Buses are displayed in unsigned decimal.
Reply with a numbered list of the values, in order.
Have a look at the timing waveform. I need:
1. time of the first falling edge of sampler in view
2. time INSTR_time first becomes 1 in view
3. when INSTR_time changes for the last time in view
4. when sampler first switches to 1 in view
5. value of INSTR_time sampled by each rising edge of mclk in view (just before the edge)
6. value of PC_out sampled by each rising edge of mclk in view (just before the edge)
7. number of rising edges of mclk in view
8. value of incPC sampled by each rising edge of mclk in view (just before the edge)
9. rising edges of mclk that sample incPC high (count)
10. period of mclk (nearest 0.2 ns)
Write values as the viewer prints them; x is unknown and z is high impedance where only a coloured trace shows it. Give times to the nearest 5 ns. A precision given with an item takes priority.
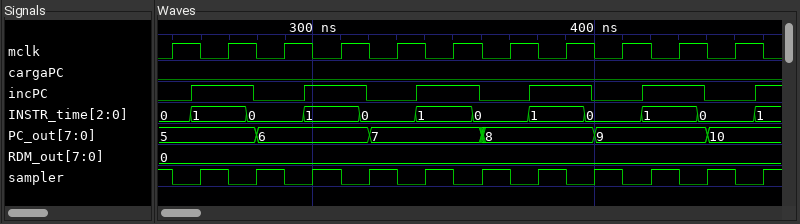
1. 250 ns
2. 255 ns
3. 455 ns
4. 260 ns
5. 0, 1, 0, 1, 0, 1, 0, 1, 0, 1, 0
6. 5, 5, 6, 6, 7, 7, 8, 8, 9, 9, 10
7. 11
8. 0 1 0 1 0 1 0 1 0 1 0
9. 5
10. 20 ns
